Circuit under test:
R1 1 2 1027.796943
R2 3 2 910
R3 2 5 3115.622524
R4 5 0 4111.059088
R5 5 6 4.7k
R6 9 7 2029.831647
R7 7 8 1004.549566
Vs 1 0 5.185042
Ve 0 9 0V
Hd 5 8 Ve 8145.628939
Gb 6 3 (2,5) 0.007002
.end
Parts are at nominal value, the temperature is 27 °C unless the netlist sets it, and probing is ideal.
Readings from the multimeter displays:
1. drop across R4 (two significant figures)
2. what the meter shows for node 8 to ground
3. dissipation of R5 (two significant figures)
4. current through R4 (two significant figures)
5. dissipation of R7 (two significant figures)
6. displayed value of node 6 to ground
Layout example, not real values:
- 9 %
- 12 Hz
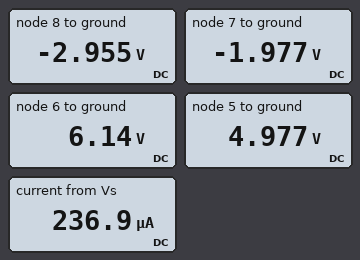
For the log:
- 5.0 V
- -2.955 V
- 290 µW
- 1.2 mA
- 950 µW
- 6.14 V
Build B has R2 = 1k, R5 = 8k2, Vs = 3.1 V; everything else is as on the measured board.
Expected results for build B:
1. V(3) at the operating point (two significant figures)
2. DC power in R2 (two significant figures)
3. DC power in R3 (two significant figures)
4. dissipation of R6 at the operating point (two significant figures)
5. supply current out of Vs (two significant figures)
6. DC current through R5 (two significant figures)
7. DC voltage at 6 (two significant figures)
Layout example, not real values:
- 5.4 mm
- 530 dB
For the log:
- 2.8 V
- 22 µW
- 140 nW
- 690 µW
- 140 µA
- 150 µA
- 4.2 V
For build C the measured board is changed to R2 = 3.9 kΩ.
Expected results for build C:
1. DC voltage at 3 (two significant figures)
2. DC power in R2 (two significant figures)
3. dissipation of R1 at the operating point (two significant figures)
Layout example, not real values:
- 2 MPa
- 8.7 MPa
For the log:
- 4.0 V
- 240 µW
- 58 µW
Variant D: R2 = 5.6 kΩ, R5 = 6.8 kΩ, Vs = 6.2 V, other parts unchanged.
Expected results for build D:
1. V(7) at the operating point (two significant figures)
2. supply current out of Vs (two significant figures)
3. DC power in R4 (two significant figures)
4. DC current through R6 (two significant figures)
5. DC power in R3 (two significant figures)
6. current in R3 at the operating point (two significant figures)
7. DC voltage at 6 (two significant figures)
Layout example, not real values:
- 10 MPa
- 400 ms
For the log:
- -2.4 V
- 280 µA
- 8.6 mW
- 1.2 mA
- 580 nW
- 14 µA
- 8.0 V
